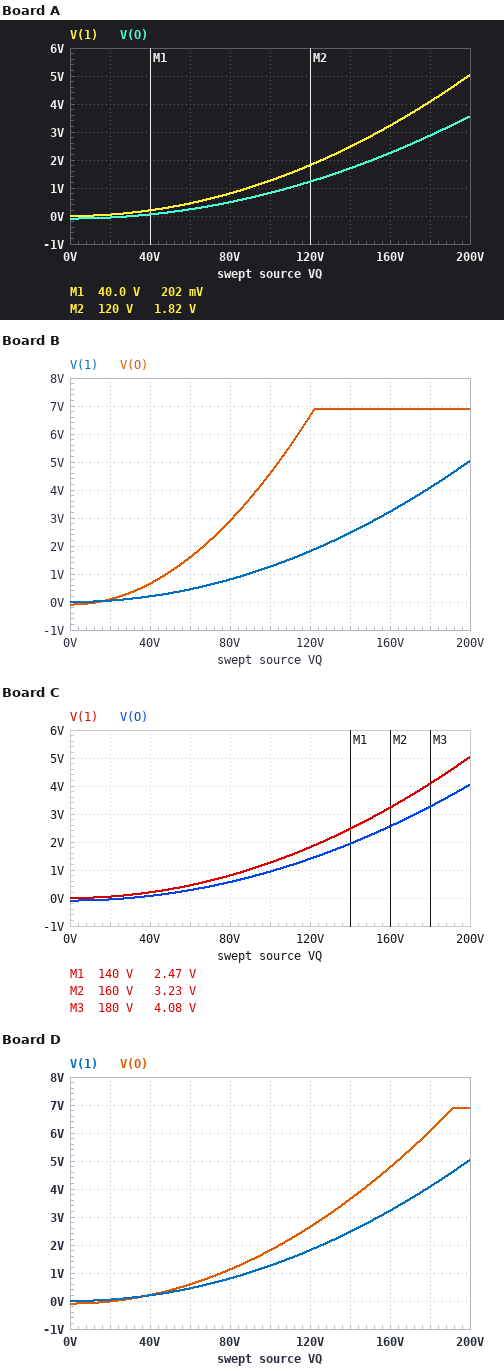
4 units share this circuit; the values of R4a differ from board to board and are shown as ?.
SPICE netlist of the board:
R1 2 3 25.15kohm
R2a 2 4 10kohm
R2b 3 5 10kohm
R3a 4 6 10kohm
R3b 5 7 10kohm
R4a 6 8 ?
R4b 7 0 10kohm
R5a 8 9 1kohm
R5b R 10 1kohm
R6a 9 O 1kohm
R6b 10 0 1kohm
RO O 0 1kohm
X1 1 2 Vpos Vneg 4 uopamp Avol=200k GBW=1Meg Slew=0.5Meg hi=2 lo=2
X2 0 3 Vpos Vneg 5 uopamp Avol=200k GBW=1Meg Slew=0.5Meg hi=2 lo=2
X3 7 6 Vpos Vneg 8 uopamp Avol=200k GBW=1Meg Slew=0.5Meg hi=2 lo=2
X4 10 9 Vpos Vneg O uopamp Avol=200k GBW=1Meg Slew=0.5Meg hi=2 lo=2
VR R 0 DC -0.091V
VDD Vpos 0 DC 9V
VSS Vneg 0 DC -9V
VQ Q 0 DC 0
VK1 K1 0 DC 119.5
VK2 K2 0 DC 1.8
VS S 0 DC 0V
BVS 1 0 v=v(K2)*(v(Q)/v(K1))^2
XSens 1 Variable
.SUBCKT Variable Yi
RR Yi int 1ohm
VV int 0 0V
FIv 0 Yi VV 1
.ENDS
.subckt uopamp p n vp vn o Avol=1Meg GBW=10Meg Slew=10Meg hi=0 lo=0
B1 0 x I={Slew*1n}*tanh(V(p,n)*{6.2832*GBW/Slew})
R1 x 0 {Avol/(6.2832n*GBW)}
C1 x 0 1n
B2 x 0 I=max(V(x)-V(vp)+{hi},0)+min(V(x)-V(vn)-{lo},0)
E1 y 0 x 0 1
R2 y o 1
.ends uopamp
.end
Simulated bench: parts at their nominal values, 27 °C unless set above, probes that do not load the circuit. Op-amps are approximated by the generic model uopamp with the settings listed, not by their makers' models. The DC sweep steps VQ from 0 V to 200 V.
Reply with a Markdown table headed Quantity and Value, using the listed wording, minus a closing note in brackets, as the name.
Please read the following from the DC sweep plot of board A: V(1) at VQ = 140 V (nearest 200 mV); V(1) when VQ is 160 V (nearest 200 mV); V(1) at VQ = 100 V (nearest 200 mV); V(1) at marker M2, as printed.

| Quantity | Value |
|---|---|
| V(1) at VQ = 140 V | 2.4 V |
| V(1) when VQ is 160 V | 3.2 V |
| V(1) at VQ = 100 V | 1.2 V |
| V(1) at marker M2, as printed | 1.82 V |
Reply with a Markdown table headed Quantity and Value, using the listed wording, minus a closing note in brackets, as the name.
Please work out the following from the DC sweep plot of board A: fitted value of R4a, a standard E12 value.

| Quantity | Value |
|---|---|
| fitted value of R4a, a standard E12 value | 3.3 kΩ |
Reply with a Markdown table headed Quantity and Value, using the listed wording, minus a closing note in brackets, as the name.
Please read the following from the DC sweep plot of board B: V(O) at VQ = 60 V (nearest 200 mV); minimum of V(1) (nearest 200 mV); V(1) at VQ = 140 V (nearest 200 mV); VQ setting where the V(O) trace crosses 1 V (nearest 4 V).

| Quantity | Value |
|---|---|
| V(O) at VQ = 60 V | 1.6 V |
| minimum of V(1) | 0 V |
| V(1) at VQ = 140 V | 2.4 V |
| VQ setting where the V(O) trace crosses 1 V | 48 V |
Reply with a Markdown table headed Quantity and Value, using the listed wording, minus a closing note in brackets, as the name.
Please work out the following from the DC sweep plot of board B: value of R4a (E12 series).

| Quantity | Value |
|---|---|
| value of R4a | 22 kΩ |
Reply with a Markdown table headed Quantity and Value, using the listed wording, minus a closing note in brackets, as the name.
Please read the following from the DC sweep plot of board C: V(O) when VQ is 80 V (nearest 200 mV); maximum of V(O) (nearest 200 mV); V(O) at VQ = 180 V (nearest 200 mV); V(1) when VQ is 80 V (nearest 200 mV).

| Quantity | Value |
|---|---|
| V(O) when VQ is 80 V | 600 mV |
| maximum of V(O) | 4.0 V |
| V(O) at VQ = 180 V | 3.2 V |
| V(1) when VQ is 80 V | 800 mV |
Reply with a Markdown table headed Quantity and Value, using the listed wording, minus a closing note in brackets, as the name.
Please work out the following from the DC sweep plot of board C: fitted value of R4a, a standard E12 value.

| Quantity | Value |
|---|---|
| fitted value of R4a, a standard E12 value | 3.9 kΩ |
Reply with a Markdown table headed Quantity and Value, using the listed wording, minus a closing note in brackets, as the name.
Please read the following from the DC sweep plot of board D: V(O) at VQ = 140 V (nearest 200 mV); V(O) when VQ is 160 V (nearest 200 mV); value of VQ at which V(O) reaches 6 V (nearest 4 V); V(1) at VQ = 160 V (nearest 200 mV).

| Quantity | Value |
|---|---|
| V(O) at VQ = 140 V | 3.6 V |
| V(O) when VQ is 160 V | 4.8 V |
| value of VQ at which V(O) reaches 6 V | 180 V |
| V(1) at VQ = 160 V | 3.2 V |
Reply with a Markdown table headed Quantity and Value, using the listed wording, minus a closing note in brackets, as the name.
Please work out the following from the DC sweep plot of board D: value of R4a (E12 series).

| Quantity | Value |
|---|---|
| value of R4a | 8.2 kΩ |
